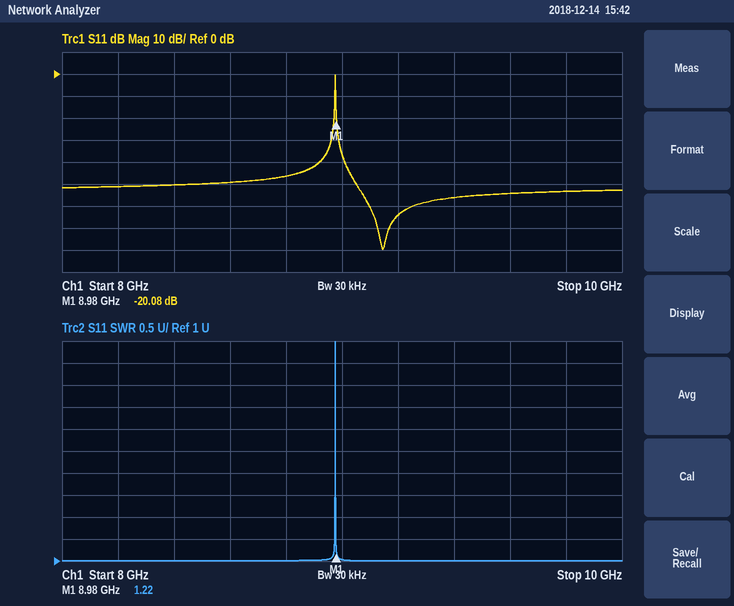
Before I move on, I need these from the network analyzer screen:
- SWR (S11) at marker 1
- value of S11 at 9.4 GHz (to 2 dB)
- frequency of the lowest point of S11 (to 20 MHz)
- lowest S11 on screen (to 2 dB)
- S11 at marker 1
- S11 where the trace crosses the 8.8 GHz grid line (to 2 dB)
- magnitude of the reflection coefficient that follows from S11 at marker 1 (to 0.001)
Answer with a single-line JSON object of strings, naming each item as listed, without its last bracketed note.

{"SWR (S11) at marker 1": "1.22", "value of S11 at 9.4 GHz": "-56 dB", "frequency of the lowest point of S11": "9.14 GHz", "lowest S11 on screen": "-80 dB", "S11 at marker 1": "-20.08 dB", "S11 where the trace crosses the 8.8 GHz grid line": "-46 dB", "magnitude of the reflection coefficient that follows from S11 at marker 1": "0.099"}
